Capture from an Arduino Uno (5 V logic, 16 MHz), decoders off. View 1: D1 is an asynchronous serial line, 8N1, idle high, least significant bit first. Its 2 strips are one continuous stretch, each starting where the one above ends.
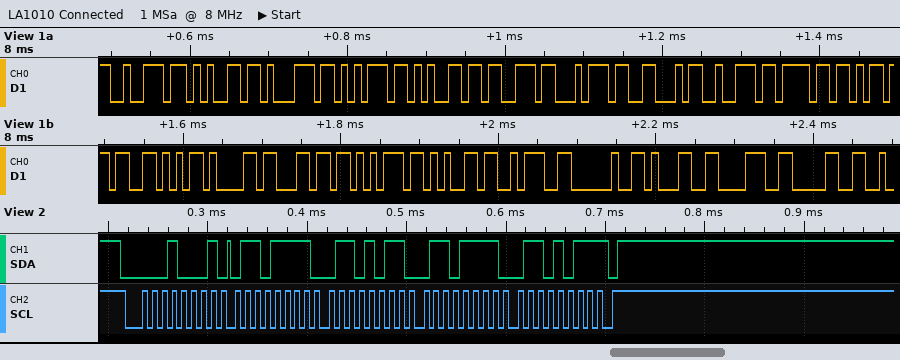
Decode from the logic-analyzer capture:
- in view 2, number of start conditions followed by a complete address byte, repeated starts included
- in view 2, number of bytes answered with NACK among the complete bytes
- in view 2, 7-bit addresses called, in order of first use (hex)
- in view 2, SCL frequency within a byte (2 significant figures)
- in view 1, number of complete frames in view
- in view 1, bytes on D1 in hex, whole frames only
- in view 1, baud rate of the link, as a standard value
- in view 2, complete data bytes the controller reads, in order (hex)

1
1
0x08
100 kHz
21
72 65 71 75 65 73 74 46 72 6F 6D 56 61 6C 75 65 3A 20 31 38 30
115200 baud
6F 6B 6F 6B
